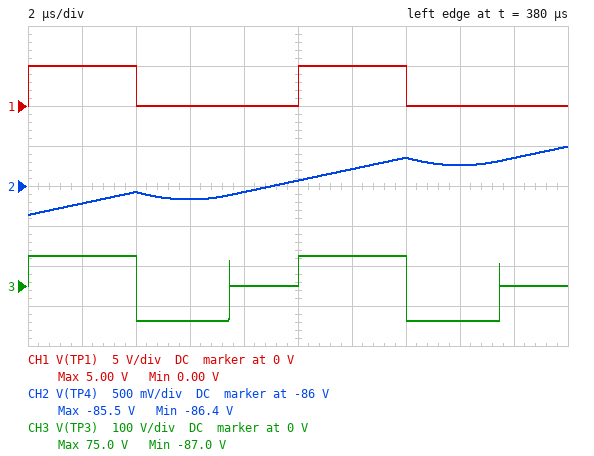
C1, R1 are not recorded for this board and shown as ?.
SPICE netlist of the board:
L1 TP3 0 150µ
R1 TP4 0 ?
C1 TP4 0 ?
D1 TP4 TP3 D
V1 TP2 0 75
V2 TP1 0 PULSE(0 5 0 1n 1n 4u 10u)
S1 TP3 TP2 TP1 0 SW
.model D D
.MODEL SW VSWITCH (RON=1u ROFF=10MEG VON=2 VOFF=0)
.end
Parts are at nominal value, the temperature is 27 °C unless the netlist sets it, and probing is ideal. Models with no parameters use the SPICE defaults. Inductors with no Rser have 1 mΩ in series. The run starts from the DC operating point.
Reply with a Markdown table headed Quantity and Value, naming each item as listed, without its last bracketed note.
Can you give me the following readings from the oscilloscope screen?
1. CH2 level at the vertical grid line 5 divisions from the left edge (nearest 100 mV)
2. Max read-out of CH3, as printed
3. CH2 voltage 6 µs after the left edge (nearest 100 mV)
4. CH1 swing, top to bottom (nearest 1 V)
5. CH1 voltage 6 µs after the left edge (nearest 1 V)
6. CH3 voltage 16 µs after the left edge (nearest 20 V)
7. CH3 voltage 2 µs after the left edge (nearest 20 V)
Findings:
| Quantity | Value |
|---|---|
| CH2 level at the vertical grid line 5 divisions from the left edge | -85.9 V |
| Max read-out of CH3, as printed | 75.0 V |
| CH2 voltage 6 µs after the left edge | -86.2 V |
| CH1 swing, top to bottom | 5 V |
| CH1 voltage 6 µs after the left edge | 0 V |
| CH3 voltage 16 µs after the left edge | -80 V |
| CH3 voltage 2 µs after the left edge | 80 V |
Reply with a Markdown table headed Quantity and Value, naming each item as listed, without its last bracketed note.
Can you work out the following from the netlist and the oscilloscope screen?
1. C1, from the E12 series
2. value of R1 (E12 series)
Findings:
| Quantity | Value |
|---|---|
| C1, from the E12 series | 12 µF |
| value of R1 | 100 Ω |
